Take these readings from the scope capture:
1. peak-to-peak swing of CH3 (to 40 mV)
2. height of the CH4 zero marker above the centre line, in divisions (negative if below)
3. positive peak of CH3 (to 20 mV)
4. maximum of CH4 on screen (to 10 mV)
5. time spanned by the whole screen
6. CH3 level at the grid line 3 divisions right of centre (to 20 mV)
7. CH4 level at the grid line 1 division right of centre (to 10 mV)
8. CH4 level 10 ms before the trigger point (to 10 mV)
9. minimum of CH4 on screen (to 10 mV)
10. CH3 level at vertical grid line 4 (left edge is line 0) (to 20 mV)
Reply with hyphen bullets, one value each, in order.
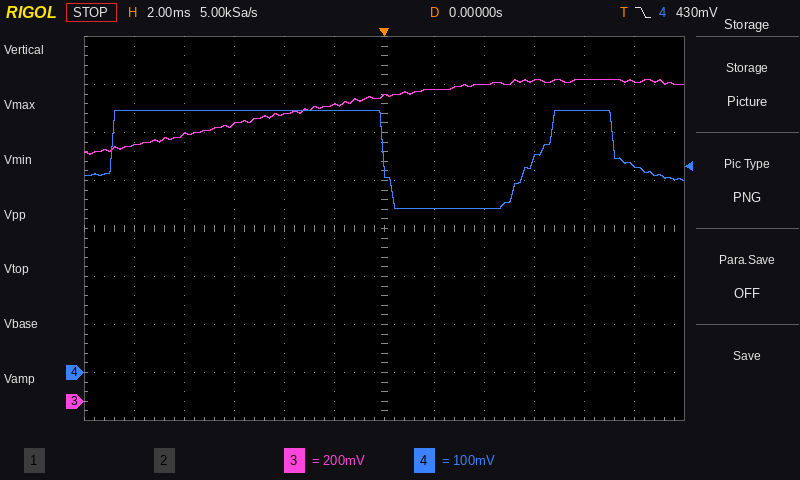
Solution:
- 320 mV
- -3.0 div
- 1.34 V
- 550 mV
- 24 ms
- 1.34 V
- 340 mV
- 550 mV
- 340 mV
- 1.20 V
